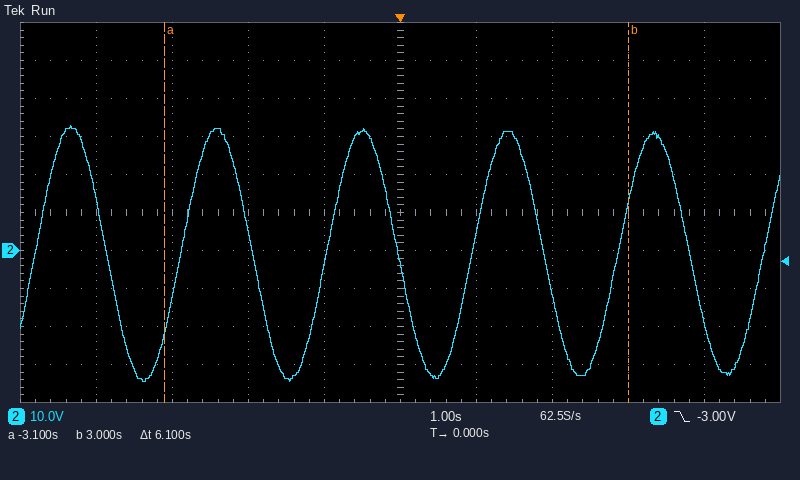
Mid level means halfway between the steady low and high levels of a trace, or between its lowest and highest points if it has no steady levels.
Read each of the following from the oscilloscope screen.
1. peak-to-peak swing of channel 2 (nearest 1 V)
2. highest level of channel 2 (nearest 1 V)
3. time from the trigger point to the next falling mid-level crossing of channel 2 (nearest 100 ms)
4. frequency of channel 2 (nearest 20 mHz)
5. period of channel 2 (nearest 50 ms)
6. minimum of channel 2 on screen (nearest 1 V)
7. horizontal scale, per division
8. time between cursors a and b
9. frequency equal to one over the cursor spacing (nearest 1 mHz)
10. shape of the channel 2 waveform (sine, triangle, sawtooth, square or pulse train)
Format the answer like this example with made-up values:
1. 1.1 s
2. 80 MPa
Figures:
1. 67 V
2. 33 V
3. 1.9 s
4. 520 mHz
5. 1.90 s
6. -34 V
7. 1 s
8. 6.1 s
9. 164 mHz
10. sine
